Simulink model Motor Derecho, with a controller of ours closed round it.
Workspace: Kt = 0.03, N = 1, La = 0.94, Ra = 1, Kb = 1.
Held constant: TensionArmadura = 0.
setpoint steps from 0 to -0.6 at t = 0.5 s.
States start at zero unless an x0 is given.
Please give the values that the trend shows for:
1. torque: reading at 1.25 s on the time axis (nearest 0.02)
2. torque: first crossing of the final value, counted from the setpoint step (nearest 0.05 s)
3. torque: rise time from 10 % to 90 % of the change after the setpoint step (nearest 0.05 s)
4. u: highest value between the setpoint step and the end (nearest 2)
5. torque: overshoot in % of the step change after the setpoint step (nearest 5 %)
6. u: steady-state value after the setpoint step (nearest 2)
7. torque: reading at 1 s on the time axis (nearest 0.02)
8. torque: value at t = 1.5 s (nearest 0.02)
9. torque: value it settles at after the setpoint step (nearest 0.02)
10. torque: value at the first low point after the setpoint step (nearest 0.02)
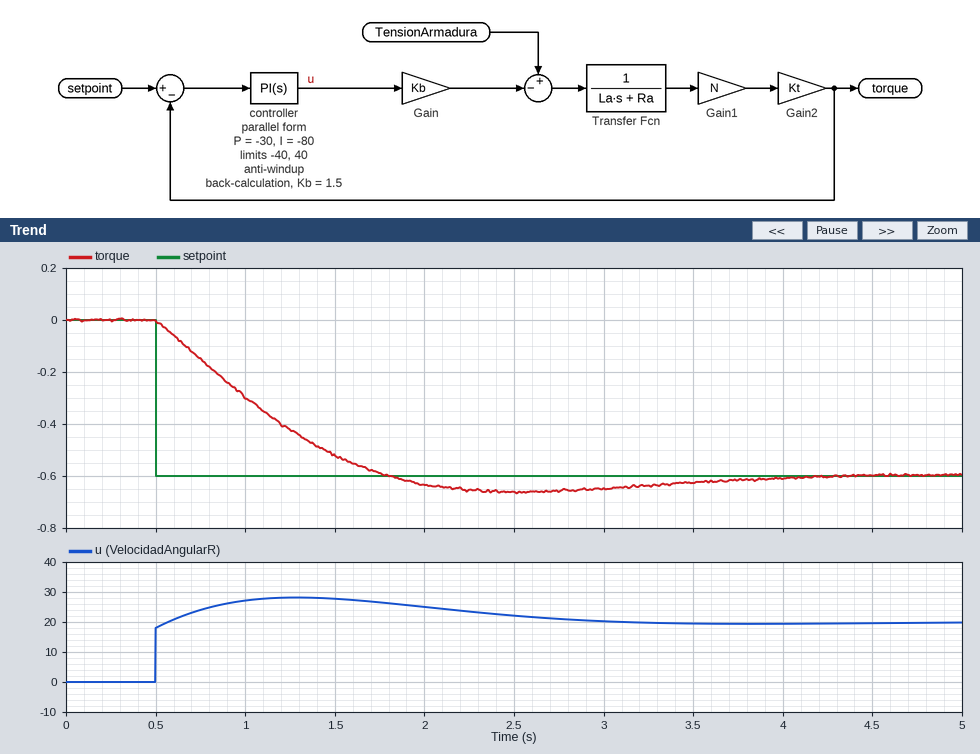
-0.42
1.30 s
0.95 s
28
10 %
20
-0.30
-0.52
-0.60
-0.66
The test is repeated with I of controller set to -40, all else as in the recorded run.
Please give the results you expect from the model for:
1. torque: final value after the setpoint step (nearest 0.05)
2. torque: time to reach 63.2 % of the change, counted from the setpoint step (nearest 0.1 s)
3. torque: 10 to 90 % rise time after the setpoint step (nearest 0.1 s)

-0.60
0.9 s
1.8 s
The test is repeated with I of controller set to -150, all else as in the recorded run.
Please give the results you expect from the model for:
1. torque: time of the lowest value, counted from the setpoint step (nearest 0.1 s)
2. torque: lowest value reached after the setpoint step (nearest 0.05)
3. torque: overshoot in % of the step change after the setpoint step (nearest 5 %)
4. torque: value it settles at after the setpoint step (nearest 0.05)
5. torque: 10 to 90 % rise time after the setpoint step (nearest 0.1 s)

1.4 s
-0.75
20 %
-0.60
0.6 s
